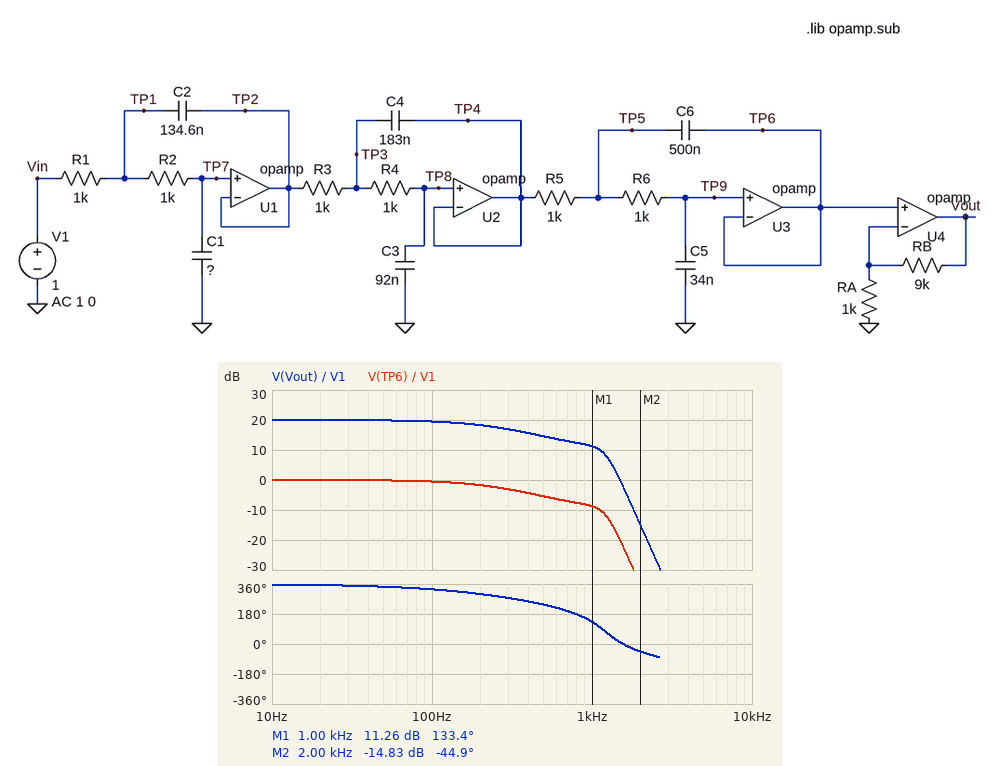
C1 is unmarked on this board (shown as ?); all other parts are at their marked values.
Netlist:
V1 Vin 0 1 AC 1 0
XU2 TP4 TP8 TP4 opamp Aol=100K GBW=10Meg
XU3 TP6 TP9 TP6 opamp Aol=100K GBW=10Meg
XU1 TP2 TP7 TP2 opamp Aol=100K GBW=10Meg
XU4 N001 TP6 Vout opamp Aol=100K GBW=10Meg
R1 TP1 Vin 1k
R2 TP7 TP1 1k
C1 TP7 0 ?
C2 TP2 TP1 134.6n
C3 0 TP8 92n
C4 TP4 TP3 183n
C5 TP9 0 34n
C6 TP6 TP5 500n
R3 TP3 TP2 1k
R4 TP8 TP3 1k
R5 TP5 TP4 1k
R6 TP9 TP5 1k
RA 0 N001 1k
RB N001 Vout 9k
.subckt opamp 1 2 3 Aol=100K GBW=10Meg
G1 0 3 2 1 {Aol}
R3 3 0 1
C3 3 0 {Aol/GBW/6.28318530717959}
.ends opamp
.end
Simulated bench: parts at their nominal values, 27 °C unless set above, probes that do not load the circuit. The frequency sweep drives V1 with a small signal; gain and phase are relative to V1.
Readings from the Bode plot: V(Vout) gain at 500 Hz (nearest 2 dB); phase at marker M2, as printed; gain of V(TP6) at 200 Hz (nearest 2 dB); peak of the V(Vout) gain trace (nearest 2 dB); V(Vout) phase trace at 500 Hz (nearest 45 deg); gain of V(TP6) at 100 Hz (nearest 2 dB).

14 dB
-44.9 deg
-2 dB
20 dB
225 deg
0 dB
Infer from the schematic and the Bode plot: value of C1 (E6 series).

330 nF
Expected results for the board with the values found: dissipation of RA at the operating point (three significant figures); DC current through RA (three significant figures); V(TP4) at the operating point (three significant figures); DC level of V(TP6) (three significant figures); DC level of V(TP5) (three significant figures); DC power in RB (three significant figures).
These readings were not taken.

1.00 mW
1.00 mA
1.00 V
1.00 V
1.00 V
9.00 mW
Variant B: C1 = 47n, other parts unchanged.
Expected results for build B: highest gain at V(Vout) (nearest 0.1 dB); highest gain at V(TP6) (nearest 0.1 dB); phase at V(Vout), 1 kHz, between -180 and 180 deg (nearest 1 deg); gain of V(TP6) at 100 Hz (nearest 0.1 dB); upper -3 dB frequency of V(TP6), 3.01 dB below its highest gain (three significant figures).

24.2 dB
4.2 dB
-165 deg
0.1 dB
1.32 kHz
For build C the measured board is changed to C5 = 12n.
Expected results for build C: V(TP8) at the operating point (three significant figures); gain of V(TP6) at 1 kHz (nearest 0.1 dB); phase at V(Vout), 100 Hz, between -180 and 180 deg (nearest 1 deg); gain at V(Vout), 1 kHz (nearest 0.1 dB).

1.00 V
-11.9 dB
-30 deg
8.1 dB
